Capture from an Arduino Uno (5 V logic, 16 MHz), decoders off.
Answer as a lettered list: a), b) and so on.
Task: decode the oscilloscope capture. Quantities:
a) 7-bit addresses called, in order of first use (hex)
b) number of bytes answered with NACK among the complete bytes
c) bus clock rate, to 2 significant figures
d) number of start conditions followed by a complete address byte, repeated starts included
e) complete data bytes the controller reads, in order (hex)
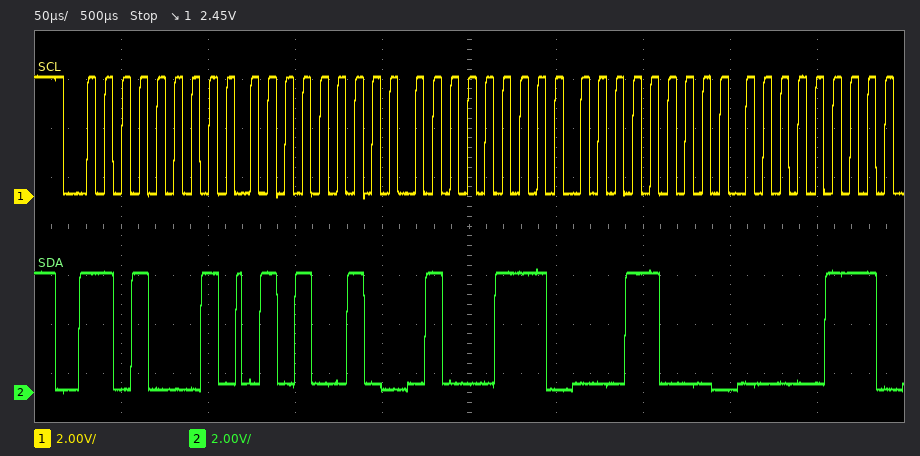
a) 0x68
b) 0
c) 100 kHz
d) 1
e) 52 47 18 07
